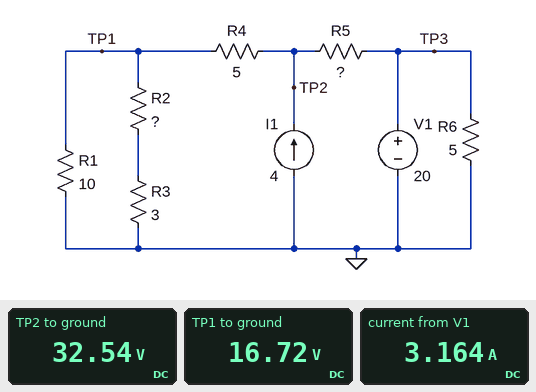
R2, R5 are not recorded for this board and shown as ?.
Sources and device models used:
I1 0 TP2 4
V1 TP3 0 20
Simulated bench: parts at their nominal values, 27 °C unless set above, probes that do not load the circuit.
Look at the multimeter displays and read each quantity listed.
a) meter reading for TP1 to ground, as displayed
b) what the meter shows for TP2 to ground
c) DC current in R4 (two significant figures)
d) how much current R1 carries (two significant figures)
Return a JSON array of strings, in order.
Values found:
["16.72 V", "32.54 V", "3.2 A", "1.7 A"]
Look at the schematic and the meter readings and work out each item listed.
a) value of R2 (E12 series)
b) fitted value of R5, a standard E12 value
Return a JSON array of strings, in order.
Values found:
["8.2 Ω", "15 Ω"]
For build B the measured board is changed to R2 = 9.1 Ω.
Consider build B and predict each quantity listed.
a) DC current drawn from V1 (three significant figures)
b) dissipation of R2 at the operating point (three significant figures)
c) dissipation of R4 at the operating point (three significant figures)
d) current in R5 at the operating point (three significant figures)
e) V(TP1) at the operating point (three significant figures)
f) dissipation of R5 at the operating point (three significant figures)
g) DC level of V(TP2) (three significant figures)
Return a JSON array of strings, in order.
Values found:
["3.14 A", "18.4 W", "49.3 W", "860 mA", "17.2 V", "11.1 W", "32.9 V"]
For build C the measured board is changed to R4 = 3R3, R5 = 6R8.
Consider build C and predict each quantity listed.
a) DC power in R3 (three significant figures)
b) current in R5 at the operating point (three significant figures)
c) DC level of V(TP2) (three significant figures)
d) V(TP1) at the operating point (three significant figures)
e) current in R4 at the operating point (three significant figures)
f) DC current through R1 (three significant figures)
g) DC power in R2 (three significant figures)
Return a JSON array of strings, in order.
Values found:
["6.28 W", "932 mA", "26.3 V", "16.2 V", "3.07 A", "1.62 A", "17.2 W"]
